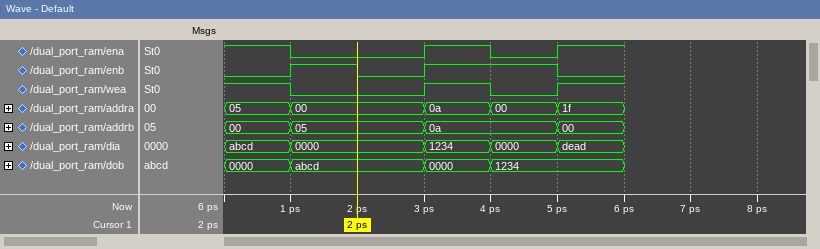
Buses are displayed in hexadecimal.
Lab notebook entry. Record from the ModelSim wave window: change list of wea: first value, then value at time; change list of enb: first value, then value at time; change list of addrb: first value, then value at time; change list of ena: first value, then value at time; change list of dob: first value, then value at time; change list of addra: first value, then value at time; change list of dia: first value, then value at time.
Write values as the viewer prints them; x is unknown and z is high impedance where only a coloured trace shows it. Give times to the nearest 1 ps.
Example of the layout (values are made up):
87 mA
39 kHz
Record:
1, 0 at 1 ps, 1 at 3 ps, 0 at 4 ps, 1 at 5 ps
0, 1 at 1 ps, 0 at 2 ps, 1 at 3 ps, 0 at 5 ps
00, 05 at 1 ps, 0a at 3 ps, 00 at 5 ps
1, 0 at 1 ps, 1 at 3 ps, 0 at 4 ps, 1 at 5 ps
0000, abcd at 1 ps, 0000 at 3 ps, 1234 at 4 ps
05, 00 at 1 ps, 0a at 3 ps, 00 at 4 ps, 1f at 5 ps
abcd, 0000 at 1 ps, 1234 at 3 ps, 0000 at 4 ps, dead at 5 ps
